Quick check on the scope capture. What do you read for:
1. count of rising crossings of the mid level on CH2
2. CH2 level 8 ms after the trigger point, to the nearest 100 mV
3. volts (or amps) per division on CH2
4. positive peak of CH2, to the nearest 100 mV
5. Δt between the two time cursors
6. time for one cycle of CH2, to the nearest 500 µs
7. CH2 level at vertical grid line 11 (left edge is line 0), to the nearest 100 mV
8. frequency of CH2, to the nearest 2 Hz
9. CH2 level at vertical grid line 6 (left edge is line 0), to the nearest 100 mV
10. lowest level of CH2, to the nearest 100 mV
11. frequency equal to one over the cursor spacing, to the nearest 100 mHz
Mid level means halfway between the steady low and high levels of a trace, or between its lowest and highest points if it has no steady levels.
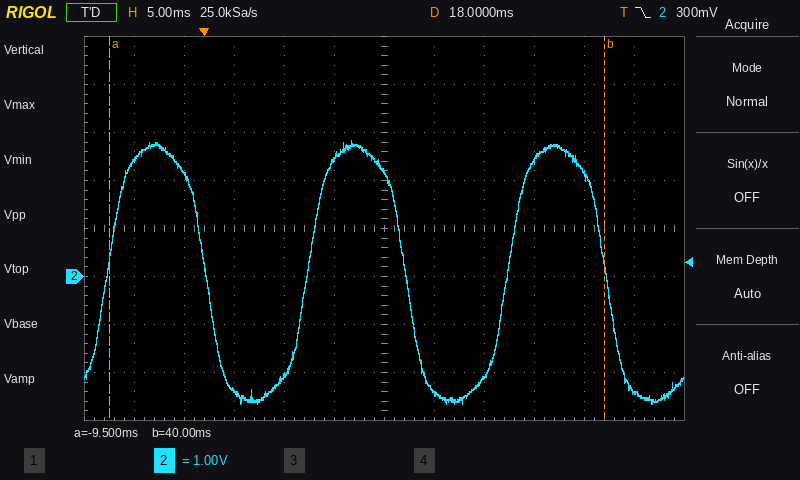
3
-2.1 V
1 V
2.8 V
49.5 ms
20.0 ms
-2.4 V
50 Hz
2.2 V
-2.6 V
20.2 Hz
